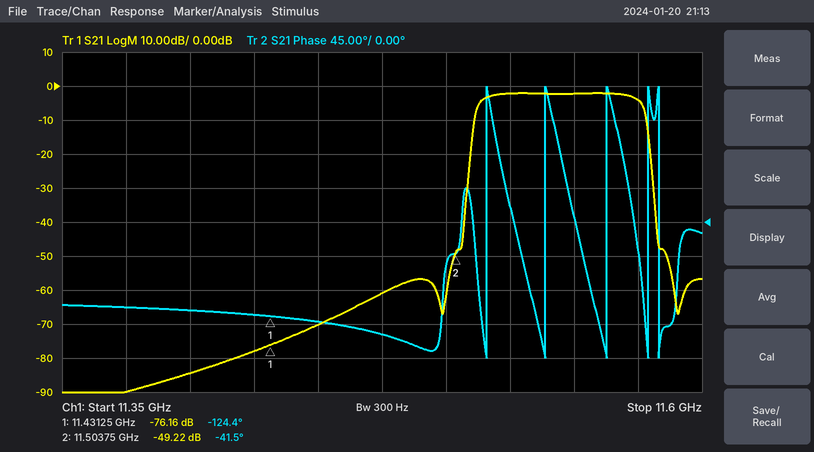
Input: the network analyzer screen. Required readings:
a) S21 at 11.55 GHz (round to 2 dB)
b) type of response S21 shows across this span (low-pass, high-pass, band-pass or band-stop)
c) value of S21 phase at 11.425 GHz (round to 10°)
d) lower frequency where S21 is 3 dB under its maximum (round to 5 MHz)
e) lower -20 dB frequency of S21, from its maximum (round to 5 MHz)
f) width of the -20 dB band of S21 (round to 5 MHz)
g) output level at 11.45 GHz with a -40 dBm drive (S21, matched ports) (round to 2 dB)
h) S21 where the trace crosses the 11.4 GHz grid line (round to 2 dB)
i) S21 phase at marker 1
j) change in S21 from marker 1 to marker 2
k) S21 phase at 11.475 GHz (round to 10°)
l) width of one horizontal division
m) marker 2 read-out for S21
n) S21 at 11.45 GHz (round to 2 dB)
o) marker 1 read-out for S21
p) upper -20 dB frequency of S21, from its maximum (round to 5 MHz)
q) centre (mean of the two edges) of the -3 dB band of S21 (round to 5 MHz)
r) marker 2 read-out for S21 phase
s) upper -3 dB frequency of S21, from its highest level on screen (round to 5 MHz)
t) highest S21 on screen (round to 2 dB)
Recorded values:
-2 dB
band-pass
-120°
11.515 GHz
11.510 GHz
70 MHz
-110 dBm
-84 dB
-124.4°
26.94 dB
-150°
25 MHz
-49.22 dB
-70 dB
-76.16 dB
11.580 GHz
11.545 GHz
-41.5°
11.575 GHz
-2 dB
